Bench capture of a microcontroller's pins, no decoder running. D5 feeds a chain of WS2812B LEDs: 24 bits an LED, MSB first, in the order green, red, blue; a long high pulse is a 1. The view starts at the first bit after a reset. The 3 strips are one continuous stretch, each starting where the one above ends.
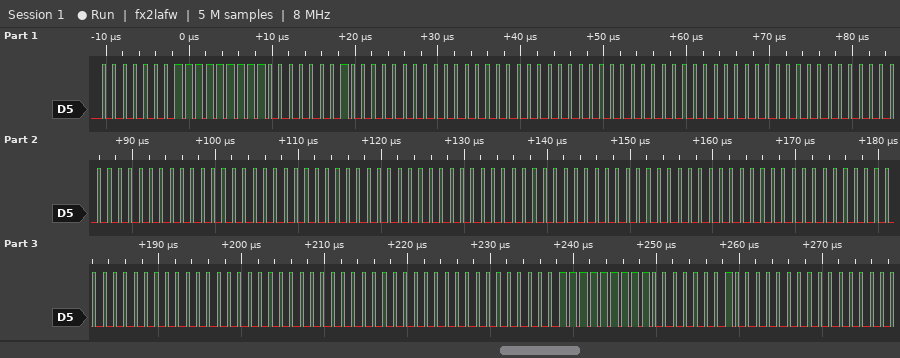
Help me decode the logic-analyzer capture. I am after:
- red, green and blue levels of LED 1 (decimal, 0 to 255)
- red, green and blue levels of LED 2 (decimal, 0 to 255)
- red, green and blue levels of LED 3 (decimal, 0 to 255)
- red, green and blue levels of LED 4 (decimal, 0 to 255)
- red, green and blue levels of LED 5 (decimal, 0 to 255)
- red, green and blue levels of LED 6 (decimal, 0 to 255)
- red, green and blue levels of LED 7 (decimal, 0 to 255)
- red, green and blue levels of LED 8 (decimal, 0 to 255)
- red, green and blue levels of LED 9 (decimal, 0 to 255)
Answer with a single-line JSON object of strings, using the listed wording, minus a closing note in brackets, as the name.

{"red, green and blue levels of LED 1": "255, 1, 1", "red, green and blue levels of LED 2": "0, 0, 0", "red, green and blue levels of LED 3": "0, 0, 0", "red, green and blue levels of LED 4": "0, 0, 0", "red, green and blue levels of LED 5": "0, 0, 0", "red, green and blue levels of LED 6": "0, 0, 0", "red, green and blue levels of LED 7": "0, 0, 0", "red, green and blue levels of LED 8": "0, 0, 0", "red, green and blue levels of LED 9": "255, 1, 1"}
